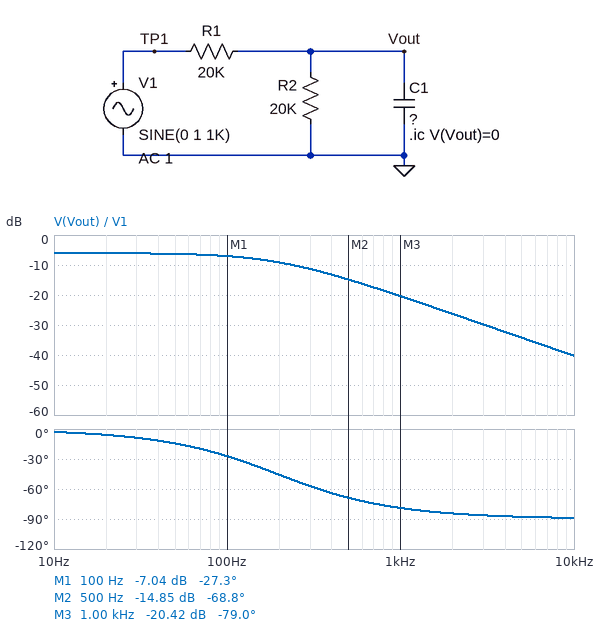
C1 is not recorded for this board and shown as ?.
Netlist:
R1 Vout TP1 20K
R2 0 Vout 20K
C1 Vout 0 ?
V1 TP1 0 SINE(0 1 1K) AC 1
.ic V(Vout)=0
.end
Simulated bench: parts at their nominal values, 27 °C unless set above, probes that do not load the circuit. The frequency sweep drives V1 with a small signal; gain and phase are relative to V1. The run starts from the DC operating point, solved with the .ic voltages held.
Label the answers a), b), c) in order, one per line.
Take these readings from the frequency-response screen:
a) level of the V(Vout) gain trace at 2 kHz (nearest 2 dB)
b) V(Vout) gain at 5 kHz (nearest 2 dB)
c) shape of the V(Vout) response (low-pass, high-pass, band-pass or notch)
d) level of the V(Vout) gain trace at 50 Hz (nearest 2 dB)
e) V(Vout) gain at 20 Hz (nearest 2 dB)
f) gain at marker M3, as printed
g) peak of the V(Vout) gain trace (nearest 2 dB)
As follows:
a) -26 dB
b) -34 dB
c) low-pass
d) -6 dB
e) -6 dB
f) -20.42 dB
g) -6 dB
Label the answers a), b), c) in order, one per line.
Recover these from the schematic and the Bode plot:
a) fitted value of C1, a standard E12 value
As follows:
a) 82 nF
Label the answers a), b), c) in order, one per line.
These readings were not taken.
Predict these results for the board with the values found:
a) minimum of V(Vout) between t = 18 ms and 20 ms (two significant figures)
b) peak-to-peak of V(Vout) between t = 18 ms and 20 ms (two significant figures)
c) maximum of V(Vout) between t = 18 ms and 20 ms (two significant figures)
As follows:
a) -95 mV
b) 190 mV
c) 95 mV
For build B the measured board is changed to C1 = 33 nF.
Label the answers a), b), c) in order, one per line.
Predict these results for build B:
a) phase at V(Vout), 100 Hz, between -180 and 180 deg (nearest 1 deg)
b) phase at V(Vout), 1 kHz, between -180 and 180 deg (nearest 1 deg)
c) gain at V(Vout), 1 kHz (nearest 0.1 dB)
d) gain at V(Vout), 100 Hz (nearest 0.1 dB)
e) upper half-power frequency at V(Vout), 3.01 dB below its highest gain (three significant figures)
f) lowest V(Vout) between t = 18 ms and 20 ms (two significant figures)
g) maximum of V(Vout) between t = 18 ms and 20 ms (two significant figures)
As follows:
a) -12 deg
b) -64 deg
c) -13.3 dB
d) -6.2 dB
e) 482 Hz
f) -220 mV
g) 220 mV
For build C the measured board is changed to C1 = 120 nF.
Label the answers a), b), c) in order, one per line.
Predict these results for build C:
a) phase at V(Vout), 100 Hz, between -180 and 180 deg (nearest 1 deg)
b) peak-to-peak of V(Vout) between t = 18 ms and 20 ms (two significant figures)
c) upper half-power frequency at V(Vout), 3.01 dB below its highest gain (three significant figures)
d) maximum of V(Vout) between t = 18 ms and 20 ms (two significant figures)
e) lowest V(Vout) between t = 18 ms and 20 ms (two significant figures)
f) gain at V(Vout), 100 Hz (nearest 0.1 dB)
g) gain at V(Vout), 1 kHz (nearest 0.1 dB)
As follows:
a) -37 deg
b) 130 mV
c) 133 Hz
d) 66 mV
e) -66 mV
f) -8.0 dB
g) -23.6 dB
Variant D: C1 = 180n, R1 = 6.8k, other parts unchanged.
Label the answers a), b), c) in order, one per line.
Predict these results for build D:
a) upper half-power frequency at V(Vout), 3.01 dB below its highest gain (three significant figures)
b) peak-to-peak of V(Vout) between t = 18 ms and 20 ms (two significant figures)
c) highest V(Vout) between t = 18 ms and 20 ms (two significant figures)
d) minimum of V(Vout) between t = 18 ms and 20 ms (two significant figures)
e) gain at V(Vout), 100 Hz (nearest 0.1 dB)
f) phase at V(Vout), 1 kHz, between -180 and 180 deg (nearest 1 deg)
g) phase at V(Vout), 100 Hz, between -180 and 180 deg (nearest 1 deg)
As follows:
a) 174 Hz
b) 260 mV
c) 130 mV
d) -130 mV
e) -3.8 dB
f) -80 deg
g) -30 deg
